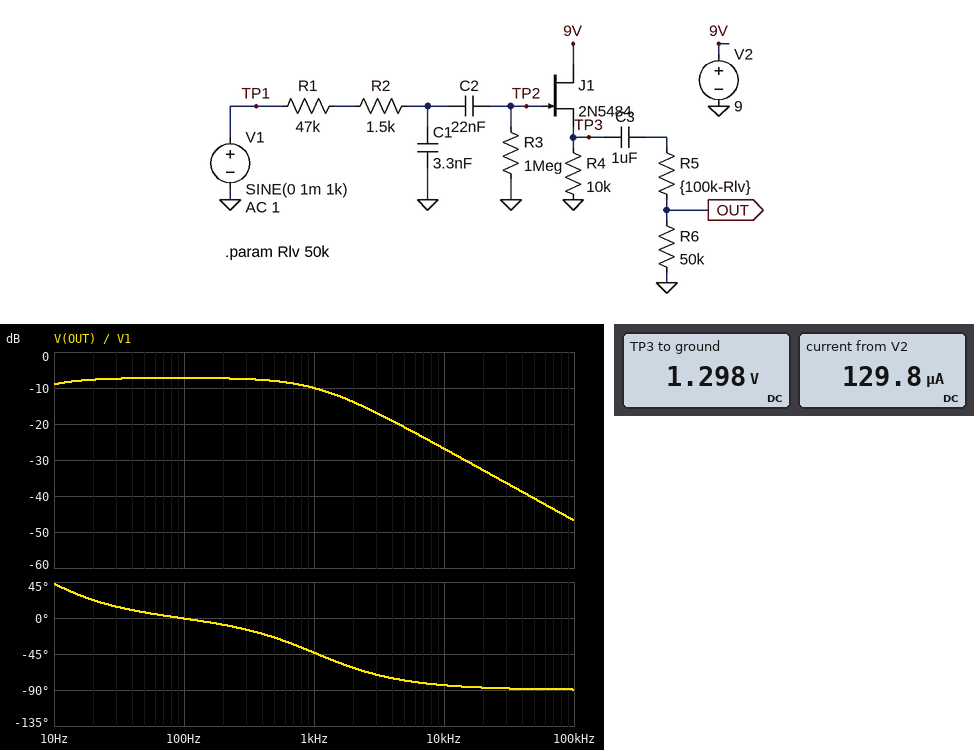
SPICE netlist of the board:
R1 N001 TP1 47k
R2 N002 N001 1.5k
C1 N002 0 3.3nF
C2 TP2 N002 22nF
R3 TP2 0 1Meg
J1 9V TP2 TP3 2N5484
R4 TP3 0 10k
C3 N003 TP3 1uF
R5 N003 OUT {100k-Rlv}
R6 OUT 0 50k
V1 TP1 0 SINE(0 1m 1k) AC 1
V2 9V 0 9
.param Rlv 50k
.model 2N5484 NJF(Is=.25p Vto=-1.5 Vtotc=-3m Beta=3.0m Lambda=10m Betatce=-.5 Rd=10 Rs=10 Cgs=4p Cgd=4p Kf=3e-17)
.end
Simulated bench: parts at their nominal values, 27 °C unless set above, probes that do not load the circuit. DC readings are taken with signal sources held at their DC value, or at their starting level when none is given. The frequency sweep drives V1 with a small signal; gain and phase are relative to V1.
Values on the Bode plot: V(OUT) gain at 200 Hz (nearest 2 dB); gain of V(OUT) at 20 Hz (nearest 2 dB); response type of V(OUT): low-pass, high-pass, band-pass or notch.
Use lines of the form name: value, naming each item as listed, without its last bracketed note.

V(OUT) gain at 200 Hz: -8 dB
gain of V(OUT) at 20 Hz: -8 dB
response type of V(OUT): low-pass, high-pass, band-pass or notch: low-pass
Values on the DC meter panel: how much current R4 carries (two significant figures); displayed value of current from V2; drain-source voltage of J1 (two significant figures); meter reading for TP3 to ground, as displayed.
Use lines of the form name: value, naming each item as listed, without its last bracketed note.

how much current R4 carries: 130 µA
displayed value of current from V2: 129.8 µA
drain-source voltage of J1: 7.7 V
meter reading for TP3 to ground, as displayed: 1.298 V
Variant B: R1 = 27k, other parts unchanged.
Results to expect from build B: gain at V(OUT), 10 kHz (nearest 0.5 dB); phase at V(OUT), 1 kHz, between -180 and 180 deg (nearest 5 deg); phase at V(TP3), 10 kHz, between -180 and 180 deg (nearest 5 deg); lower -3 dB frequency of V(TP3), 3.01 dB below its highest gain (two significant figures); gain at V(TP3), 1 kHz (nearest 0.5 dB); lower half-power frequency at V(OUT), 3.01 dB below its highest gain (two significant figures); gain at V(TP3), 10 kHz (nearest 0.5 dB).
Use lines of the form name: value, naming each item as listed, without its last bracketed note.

gain at V(OUT), 10 kHz: -22.5 dB
phase at V(OUT), 1 kHz, between -180 and 180 deg: -30 deg
phase at V(TP3), 10 kHz, between -180 and 180 deg: -80 deg
lower -3 dB frequency of V(TP3), 3.01 dB below its highest gain: 7.0 Hz
gain at V(TP3), 1 kHz: -2.0 dB
lower half-power frequency at V(OUT), 3.01 dB below its highest gain: 7.3 Hz
gain at V(TP3), 10 kHz: -16.5 dB
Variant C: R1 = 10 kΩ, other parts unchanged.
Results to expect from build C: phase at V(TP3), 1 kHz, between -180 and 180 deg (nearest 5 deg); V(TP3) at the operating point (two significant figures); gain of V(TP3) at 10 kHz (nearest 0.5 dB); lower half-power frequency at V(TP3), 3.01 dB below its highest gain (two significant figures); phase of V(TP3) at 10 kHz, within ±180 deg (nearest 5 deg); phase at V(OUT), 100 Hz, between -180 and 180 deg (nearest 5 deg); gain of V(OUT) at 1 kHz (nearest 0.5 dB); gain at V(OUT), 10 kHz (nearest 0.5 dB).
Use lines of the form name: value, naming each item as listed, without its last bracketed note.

phase at V(TP3), 1 kHz, between -180 and 180 deg: -15 deg
V(TP3) at the operating point: 1.3 V
gain of V(TP3) at 10 kHz: -9.0 dB
lower half-power frequency at V(TP3), 3.01 dB below its highest gain: 7.1 Hz
phase of V(TP3) at 10 kHz, within ±180 deg: -65 deg
phase at V(OUT), 100 Hz, between -180 and 180 deg: 5 deg
gain of V(OUT) at 1 kHz: -7.0 dB
gain at V(OUT), 10 kHz: -15.0 dB
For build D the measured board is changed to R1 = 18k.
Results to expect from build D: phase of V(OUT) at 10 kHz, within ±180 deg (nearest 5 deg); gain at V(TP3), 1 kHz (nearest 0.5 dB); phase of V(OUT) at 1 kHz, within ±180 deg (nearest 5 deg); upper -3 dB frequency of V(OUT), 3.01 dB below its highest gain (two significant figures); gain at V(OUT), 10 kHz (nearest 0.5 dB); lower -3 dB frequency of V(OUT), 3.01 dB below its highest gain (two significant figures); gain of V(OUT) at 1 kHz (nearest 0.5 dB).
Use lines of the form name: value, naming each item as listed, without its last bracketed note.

phase of V(OUT) at 10 kHz, within ±180 deg: -75 deg
gain at V(TP3), 1 kHz: -1.5 dB
phase of V(OUT) at 1 kHz, within ±180 deg: -20 deg
upper -3 dB frequency of V(OUT), 3.01 dB below its highest gain: 2.5 kHz
gain at V(OUT), 10 kHz: -19.0 dB
lower -3 dB frequency of V(OUT), 3.01 dB below its highest gain: 7.4 Hz
gain of V(OUT) at 1 kHz: -7.5 dB
